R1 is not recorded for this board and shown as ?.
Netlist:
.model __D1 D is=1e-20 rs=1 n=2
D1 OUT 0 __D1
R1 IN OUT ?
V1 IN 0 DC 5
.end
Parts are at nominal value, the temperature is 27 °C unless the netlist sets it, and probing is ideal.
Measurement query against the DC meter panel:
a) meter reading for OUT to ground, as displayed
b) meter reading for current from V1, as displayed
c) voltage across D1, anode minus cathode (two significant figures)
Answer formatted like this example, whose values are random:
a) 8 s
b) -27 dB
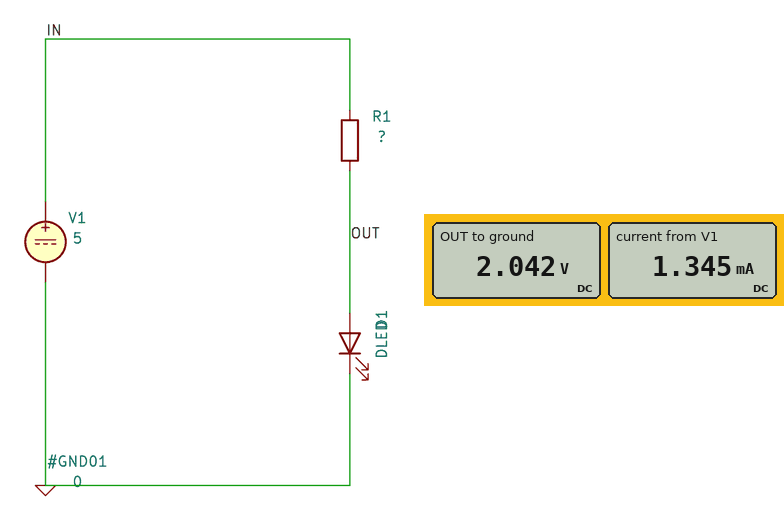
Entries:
a) 2.042 V
b) 1.345 mA
c) 2.0 V
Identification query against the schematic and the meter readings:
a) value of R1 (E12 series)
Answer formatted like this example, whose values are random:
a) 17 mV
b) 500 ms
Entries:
a) 2.2 kΩ
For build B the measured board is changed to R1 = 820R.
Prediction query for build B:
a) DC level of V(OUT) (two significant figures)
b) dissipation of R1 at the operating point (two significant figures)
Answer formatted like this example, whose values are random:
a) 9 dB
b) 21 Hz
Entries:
a) 2.1 V
b) 10 mW
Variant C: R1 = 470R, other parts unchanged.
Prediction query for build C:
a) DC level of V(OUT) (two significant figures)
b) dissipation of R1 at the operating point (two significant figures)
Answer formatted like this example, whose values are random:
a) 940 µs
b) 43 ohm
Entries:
a) 2.1 V
b) 18 mW
